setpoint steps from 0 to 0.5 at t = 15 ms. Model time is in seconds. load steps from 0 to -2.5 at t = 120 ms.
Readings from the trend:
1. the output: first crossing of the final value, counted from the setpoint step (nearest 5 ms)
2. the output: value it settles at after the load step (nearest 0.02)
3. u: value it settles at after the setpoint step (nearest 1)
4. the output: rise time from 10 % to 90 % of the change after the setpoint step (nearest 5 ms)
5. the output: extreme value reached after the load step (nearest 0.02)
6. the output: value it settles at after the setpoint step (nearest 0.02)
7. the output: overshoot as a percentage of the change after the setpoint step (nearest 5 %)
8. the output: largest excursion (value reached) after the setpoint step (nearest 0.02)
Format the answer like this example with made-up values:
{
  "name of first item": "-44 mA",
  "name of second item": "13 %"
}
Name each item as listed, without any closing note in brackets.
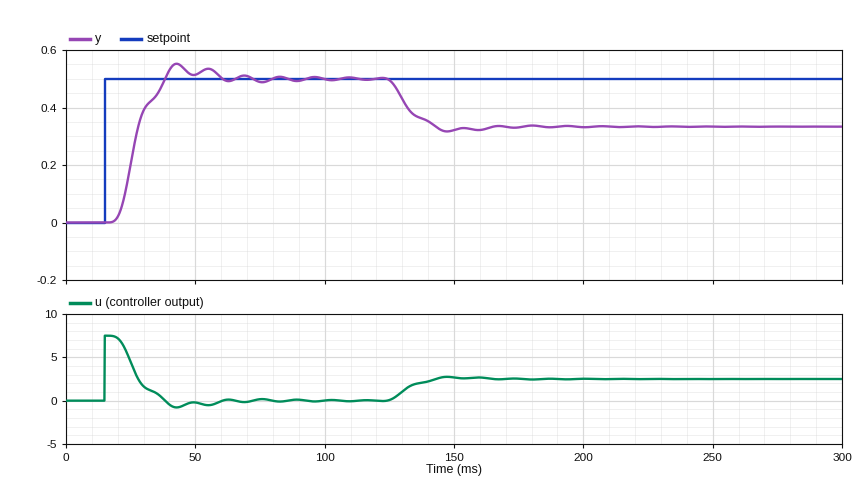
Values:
{
  "the output: first crossing of the final value, counted from the setpoint step": "25 ms",
  "the output: value it settles at after the load step": "0.34",
  "u: value it settles at after the setpoint step": "0",
  "the output: rise time from 10 % to 90 % of the change after the setpoint step": "15 ms",
  "the output: extreme value reached after the load step": "0.32",
  "the output: value it settles at after the setpoint step": "0.50",
  "the output: overshoot as a percentage of the change after the setpoint step": "10 %",
  "the output: largest excursion (value reached) after the setpoint step": "0.56"
}
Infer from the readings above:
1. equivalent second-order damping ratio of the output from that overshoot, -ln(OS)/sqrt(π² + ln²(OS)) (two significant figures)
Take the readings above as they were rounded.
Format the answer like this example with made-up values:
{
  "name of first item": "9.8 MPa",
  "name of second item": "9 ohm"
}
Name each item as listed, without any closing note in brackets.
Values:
{
  "equivalent second-order damping ratio of the output from that overshoot, -ln(OS)/sqrt(π² + ln²(OS))": "0.59"
}
